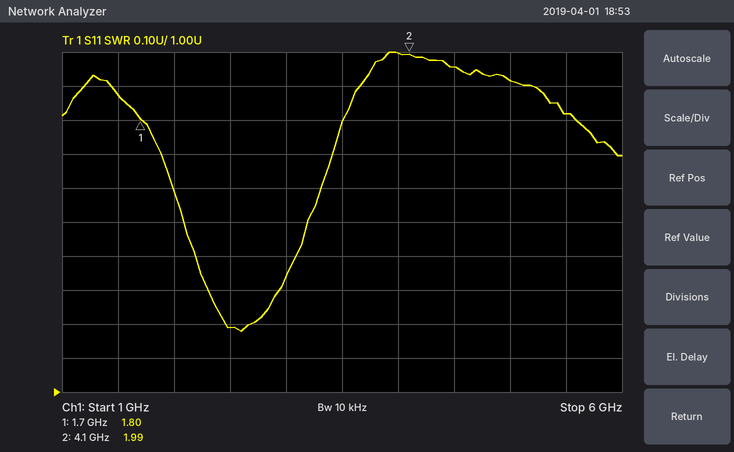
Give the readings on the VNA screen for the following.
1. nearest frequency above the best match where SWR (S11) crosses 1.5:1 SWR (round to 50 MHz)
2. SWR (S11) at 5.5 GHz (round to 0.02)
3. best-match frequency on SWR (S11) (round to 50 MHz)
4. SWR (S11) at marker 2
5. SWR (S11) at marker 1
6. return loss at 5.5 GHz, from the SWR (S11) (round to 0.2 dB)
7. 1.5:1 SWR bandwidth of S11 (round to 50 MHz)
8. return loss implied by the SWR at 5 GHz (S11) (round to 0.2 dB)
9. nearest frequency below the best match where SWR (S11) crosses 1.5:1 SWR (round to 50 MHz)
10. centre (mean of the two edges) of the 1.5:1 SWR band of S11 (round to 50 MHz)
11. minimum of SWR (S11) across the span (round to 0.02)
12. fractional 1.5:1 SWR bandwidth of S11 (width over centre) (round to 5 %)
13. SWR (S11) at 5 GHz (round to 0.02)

3.20 GHz
1.82
2.60 GHz
1.99
1.80
10.8 dB
1.10 GHz
10.0 dB
2.10 GHz
2.65 GHz
1.18
40 %
1.92
